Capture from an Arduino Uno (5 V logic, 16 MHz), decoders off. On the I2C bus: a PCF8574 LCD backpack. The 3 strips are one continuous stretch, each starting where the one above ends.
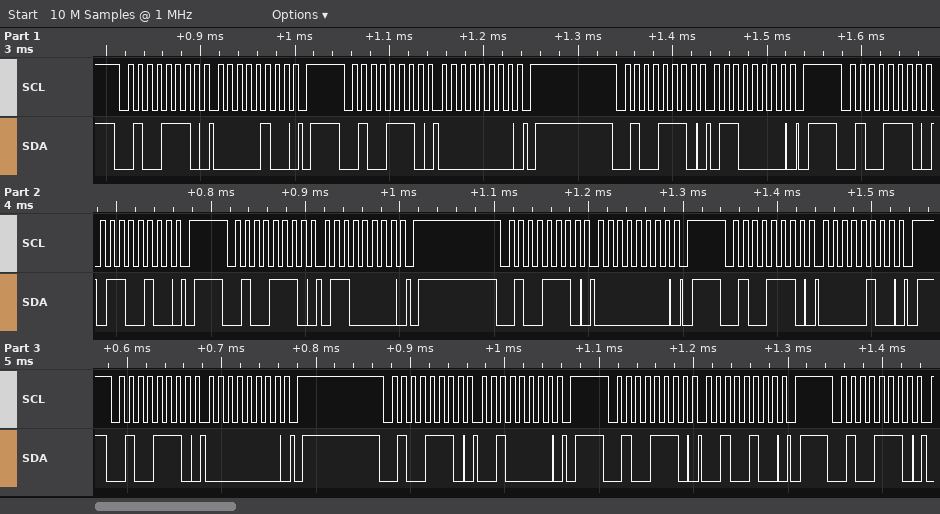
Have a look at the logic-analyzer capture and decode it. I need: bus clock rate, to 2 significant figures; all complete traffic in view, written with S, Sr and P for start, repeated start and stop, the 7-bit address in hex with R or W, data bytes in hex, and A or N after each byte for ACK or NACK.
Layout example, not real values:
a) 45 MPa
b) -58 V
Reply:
a) 100 kHz
b) S 27W A 04 A P S 27W A 00 A P S 27W A 60 A P S 27W A 64 A P S 27W A 60 A P S 27W A 00 A P S 27W A 04 A P S 27W A 00 A P S 27W A 20 A P S 27W A 24 A P S 27W A
